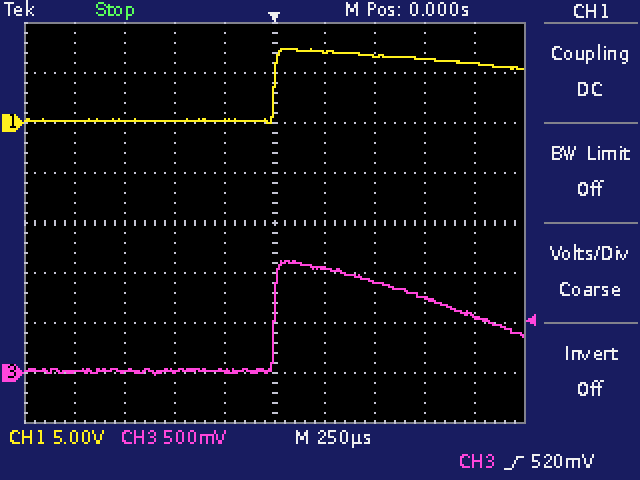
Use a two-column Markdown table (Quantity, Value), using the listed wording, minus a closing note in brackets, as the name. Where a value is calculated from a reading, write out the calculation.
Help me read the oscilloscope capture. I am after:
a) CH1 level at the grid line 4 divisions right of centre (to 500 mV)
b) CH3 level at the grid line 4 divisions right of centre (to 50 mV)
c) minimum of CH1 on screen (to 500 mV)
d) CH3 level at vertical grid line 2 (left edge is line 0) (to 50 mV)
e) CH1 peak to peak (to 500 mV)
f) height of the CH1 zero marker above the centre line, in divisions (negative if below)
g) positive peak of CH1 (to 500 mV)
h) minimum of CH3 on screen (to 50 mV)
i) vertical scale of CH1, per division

| Quantity | Value |
|---|---|
| CH1 level at the grid line 4 divisions right of centre | 6.0 V |
| CH3 level at the grid line 4 divisions right of centre | 550 mV |
| minimum of CH1 on screen | 0.0 V |
| CH3 level at vertical grid line 2 (left edge is line 0) | 0 mV |
| CH1 peak to peak | 7.5 V − (0.0 V) = 7.5 V |
| height of the CH1 zero marker above the centre line, in divisions | +2.0 div |
| positive peak of CH1 | 7.5 V |
| minimum of CH3 on screen | 0 mV |
| vertical scale of CH1, per division | 5 V |
